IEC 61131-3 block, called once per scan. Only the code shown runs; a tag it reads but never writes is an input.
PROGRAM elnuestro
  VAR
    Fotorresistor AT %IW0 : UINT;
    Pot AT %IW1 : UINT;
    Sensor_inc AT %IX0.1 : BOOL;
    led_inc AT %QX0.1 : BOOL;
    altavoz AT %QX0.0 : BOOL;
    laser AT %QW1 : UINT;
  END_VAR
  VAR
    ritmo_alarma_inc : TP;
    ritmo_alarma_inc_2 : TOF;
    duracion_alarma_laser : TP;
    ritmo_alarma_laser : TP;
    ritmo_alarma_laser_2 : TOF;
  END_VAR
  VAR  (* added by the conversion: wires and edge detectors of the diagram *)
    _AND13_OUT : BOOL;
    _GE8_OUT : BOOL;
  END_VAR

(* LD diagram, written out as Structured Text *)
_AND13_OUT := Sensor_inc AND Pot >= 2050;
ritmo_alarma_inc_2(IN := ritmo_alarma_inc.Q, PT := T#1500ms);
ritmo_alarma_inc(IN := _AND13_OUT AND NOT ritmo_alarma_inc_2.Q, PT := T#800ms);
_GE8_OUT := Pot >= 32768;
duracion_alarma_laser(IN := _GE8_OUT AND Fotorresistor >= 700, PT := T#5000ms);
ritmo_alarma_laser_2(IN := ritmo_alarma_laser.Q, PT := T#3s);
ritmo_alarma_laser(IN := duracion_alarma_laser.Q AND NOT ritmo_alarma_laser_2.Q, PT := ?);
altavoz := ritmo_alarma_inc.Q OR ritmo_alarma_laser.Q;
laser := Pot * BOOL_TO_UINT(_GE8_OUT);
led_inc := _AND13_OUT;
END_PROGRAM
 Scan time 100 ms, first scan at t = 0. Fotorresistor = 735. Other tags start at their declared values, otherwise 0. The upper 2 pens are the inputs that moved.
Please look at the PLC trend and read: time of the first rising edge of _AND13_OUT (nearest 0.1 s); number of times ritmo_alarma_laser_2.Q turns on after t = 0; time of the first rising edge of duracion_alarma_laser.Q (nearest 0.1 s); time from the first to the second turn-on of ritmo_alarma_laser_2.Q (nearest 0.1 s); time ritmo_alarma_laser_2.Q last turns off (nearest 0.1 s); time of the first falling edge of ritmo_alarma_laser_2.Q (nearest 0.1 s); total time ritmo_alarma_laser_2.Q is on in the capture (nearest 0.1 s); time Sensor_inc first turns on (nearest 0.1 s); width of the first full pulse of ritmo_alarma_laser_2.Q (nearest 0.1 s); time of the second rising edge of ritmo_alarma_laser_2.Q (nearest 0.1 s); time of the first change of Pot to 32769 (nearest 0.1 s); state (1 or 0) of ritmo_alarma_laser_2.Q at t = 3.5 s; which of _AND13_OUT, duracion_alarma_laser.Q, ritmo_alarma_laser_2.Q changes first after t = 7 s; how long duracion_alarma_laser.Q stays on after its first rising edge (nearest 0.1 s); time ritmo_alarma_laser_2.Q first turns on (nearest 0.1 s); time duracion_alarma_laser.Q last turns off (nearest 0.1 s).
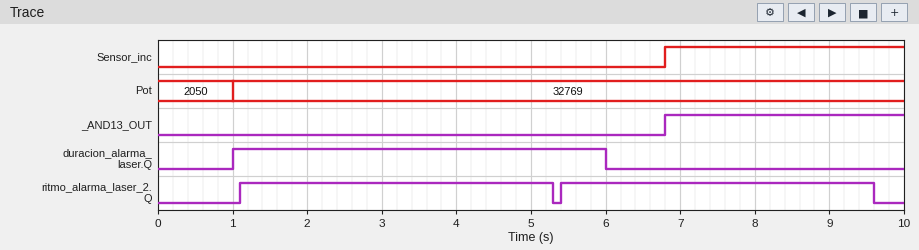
6.8 s
2
1.0 s
4.3 s
9.6 s
5.3 s
8.4 s
6.8 s
4.2 s
5.4 s
1.0 s
1
ritmo_alarma_laser_2.Q
5.0 s
1.1 s
6.0 s
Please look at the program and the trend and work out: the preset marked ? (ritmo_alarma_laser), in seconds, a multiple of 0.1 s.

1.2 s
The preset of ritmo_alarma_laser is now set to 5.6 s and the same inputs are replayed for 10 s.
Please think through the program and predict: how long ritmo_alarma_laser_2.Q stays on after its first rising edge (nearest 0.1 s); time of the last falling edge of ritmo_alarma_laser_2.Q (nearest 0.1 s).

8.6 s
9.7 s
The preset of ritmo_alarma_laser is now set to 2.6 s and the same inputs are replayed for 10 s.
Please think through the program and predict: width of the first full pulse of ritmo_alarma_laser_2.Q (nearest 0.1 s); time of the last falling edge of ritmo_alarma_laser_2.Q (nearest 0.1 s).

5.6 s
6.7 s
